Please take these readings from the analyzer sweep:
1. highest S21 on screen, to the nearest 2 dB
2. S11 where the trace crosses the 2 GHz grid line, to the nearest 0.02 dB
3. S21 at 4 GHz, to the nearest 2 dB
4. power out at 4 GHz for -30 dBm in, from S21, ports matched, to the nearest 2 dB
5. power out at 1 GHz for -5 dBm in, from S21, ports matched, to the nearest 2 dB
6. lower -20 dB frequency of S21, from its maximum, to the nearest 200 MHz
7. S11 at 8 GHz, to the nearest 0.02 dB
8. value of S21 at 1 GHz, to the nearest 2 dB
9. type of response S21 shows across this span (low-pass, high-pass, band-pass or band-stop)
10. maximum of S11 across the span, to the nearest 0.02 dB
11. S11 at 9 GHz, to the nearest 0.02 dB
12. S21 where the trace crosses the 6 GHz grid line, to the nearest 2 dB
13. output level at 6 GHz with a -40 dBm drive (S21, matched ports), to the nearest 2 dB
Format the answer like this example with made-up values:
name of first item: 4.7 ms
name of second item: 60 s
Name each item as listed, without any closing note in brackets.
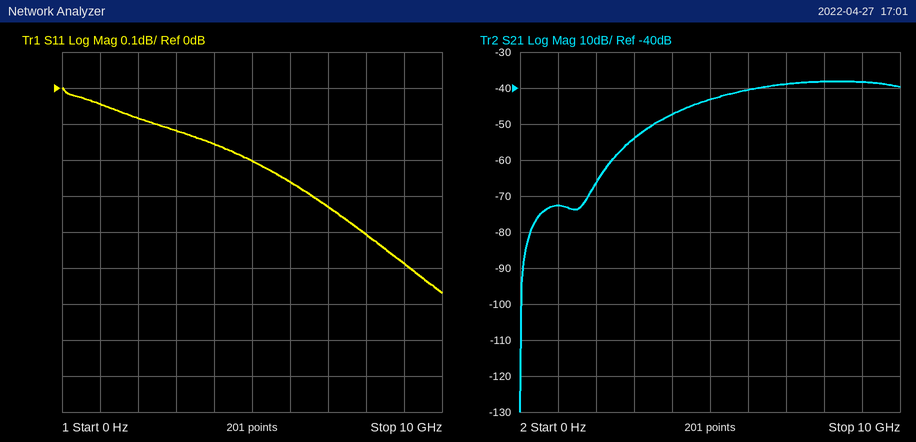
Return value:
highest S21 on screen, to the nearest 2 dB: -38 dB
S11 where the trace crosses the 2 GHz grid line, to the nearest 0.02 dB: -0.08 dB
S21 at 4 GHz, to the nearest 2 dB: -48 dB
power out at 4 GHz for -30 dBm in, from S21, ports matched, to the nearest 2 dB: -78 dBm
power out at 1 GHz for -5 dBm in, from S21, ports matched, to the nearest 2 dB: -78 dBm
lower -20 dB frequency of S21, from its maximum, to the nearest 200 MHz: 2.6 GHz
S11 at 8 GHz, to the nearest 0.02 dB: -0.40 dB
value of S21 at 1 GHz, to the nearest 2 dB: -72 dB
type of response S21 shows across this span: high-pass
maximum of S11 across the span, to the nearest 0.02 dB: 0.00 dB
S11 at 9 GHz, to the nearest 0.02 dB: -0.48 dB
S21 where the trace crosses the 6 GHz grid line, to the nearest 2 dB: -40 dB
output level at 6 GHz with a -40 dBm drive (S21, matched ports), to the nearest 2 dB: -80 dBm
